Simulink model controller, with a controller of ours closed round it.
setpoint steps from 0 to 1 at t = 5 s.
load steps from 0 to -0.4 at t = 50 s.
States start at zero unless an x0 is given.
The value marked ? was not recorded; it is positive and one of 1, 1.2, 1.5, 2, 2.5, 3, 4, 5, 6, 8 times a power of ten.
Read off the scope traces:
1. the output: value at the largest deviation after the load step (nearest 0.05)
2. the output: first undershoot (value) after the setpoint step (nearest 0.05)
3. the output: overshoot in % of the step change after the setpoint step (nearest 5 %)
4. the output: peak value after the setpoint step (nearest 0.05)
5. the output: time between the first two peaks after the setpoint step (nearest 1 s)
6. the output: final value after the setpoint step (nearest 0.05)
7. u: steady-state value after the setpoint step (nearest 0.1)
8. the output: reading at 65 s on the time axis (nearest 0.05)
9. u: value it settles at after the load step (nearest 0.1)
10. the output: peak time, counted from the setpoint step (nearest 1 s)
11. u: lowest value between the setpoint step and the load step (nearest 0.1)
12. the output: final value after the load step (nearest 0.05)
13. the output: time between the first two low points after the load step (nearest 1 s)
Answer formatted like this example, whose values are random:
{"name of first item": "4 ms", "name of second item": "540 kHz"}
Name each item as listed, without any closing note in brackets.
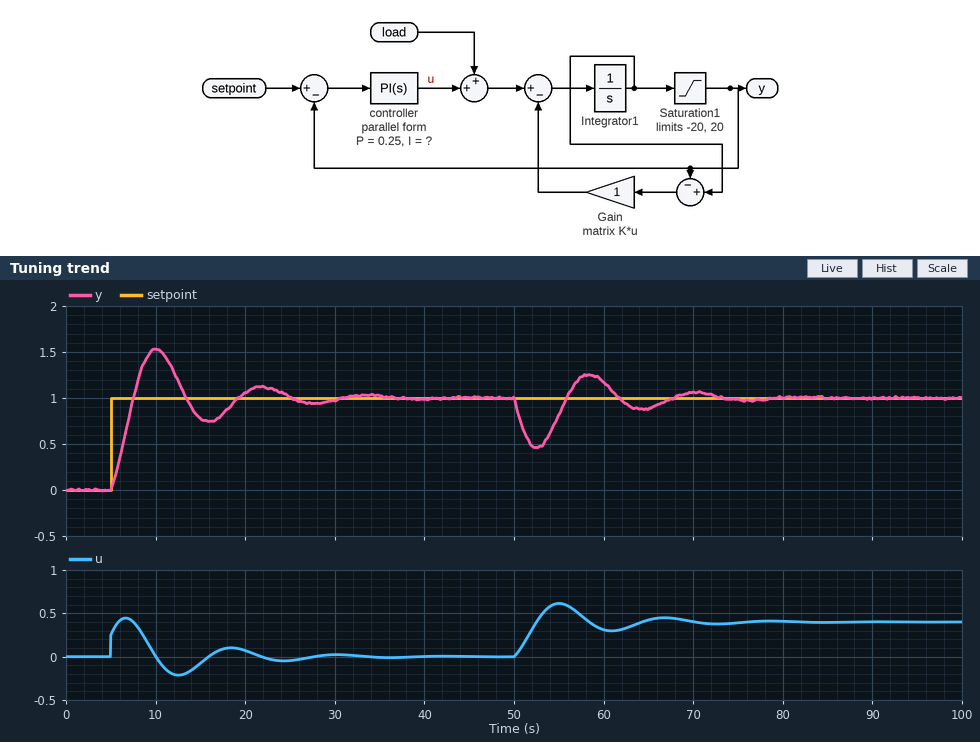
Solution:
{"the output: value at the largest deviation after the load step": "0.45", "the output: first undershoot (value) after the setpoint step": "0.75", "the output: overshoot in % of the step change after the setpoint step": "55 %", "the output: peak value after the setpoint step": "1.55", "the output: time between the first two peaks after the setpoint step": "12 s", "the output: final value after the setpoint step": "1.00", "u: steady-state value after the setpoint step": "0.0", "the output: reading at 65 s on the time axis": "0.90", "u: value it settles at after the load step": "0.4", "the output: peak time, counted from the setpoint step": "5 s", "u: lowest value between the setpoint step and the load step": "-0.2", "the output: final value after the load step": "1.00", "the output: time between the first two low points after the load step": "12 s"}
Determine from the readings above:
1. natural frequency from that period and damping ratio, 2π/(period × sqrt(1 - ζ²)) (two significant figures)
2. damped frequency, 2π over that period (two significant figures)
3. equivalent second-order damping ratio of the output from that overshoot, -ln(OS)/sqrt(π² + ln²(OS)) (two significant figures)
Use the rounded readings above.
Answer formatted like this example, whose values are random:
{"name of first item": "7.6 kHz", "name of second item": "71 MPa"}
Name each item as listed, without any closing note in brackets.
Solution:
{"natural frequency from that period and damping ratio, 2π/(period × sqrt(1 - ζ²))": "0.53 rad/s", "damped frequency, 2π over that period": "0.52 rad/s", "equivalent second-order damping ratio of the output from that overshoot, -ln(OS)/sqrt(π² + ln²(OS))": "0.19"}
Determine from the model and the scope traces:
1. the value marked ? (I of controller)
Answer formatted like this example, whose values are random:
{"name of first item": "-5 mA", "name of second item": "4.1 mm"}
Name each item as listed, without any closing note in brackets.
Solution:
{"the value marked ?": "0.3"}
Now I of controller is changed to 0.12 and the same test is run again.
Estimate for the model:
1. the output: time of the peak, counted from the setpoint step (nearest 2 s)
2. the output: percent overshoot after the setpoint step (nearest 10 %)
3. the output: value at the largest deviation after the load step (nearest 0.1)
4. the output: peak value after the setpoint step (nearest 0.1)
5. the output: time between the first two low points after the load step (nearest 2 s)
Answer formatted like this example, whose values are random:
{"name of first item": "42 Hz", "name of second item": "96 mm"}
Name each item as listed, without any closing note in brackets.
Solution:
{"the output: time of the peak, counted from the setpoint step": "8 s", "the output: percent overshoot after the setpoint step": "40 %", "the output: value at the largest deviation after the load step": "0.3", "the output: peak value after the setpoint step": "1.4", "the output: time between the first two low points after the load step": "20 s"}
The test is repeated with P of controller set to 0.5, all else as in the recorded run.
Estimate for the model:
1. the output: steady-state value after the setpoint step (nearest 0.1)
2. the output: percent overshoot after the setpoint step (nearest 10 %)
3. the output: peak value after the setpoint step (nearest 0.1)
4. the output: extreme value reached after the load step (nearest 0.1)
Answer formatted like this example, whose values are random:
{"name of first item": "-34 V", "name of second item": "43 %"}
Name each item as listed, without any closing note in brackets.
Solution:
{"the output: steady-state value after the setpoint step": "1.0", "the output: percent overshoot after the setpoint step": "30 %", "the output: peak value after the setpoint step": "1.3", "the output: extreme value reached after the load step": "0.6"}
